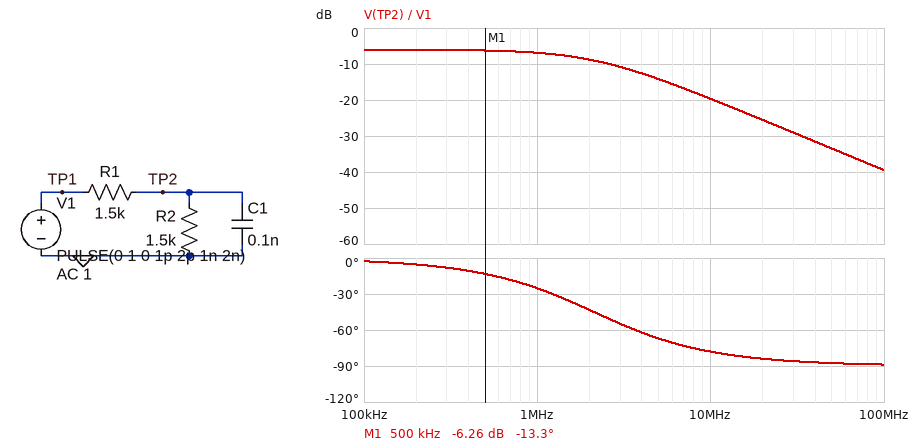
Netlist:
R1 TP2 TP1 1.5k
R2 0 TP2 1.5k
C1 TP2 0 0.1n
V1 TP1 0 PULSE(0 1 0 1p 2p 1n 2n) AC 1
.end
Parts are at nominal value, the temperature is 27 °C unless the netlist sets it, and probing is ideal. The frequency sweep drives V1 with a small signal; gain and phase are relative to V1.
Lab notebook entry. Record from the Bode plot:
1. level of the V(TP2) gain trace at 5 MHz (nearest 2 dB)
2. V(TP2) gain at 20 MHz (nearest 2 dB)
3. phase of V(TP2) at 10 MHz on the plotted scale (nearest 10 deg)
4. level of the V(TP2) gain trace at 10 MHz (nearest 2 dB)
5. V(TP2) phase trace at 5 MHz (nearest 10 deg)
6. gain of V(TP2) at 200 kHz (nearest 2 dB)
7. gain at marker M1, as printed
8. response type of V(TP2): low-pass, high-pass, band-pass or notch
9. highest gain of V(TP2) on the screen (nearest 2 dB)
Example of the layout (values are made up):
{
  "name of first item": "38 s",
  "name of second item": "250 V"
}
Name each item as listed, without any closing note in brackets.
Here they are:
{
  "level of the V(TP2) gain trace at 5 MHz": "-14 dB",
  "V(TP2) gain at 20 MHz": "-26 dB",
  "phase of V(TP2) at 10 MHz on the plotted scale": "-80 deg",
  "level of the V(TP2) gain trace at 10 MHz": "-20 dB",
  "V(TP2) phase trace at 5 MHz": "-70 deg",
  "gain of V(TP2) at 200 kHz": "-6 dB",
  "gain at marker M1, as printed": "-6.26 dB",
  "response type of V(TP2): low-pass, high-pass, band-pass or notch": "low-pass",
  "highest gain of V(TP2) on the screen": "-6 dB"
}
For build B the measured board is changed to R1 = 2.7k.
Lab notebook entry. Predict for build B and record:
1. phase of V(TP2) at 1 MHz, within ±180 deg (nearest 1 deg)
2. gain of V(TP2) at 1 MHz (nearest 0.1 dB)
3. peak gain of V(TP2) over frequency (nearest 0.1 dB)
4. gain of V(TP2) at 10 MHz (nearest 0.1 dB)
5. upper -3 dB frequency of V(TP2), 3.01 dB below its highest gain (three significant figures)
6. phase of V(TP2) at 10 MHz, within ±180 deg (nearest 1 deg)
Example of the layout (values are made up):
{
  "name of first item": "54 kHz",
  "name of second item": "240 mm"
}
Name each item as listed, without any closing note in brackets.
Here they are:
{
  "phase of V(TP2) at 1 MHz, within ±180 deg": "-31 deg",
  "gain of V(TP2) at 1 MHz": "-10.3 dB",
  "peak gain of V(TP2) over frequency": "-8.9 dB",
  "gain of V(TP2) at 10 MHz": "-24.7 dB",
  "upper -3 dB frequency of V(TP2), 3.01 dB below its highest gain": "1.65 MHz",
  "phase of V(TP2) at 10 MHz, within ±180 deg": "-81 deg"
}
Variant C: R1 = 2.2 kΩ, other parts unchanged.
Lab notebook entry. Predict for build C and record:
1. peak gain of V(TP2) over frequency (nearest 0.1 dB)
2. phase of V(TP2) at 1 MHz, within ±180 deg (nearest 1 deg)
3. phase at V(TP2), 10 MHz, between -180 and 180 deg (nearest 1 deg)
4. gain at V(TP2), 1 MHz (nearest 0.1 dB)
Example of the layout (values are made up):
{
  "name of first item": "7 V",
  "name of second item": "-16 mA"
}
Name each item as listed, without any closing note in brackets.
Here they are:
{
  "peak gain of V(TP2) over frequency": "-7.8 dB",
  "phase of V(TP2) at 1 MHz, within ±180 deg": "-29 deg",
  "phase at V(TP2), 10 MHz, between -180 and 180 deg": "-80 deg",
  "gain at V(TP2), 1 MHz": "-9.0 dB"
}
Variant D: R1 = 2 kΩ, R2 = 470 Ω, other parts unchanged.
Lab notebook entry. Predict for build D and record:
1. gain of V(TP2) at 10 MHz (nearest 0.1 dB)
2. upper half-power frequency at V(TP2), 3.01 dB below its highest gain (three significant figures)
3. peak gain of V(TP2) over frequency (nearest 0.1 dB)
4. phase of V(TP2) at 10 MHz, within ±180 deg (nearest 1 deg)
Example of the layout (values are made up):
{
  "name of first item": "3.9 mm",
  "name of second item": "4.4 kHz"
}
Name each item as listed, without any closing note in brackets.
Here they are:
{
  "gain of V(TP2) at 10 MHz": "-22.7 dB",
  "upper half-power frequency at V(TP2), 3.01 dB below its highest gain": "4.18 MHz",
  "peak gain of V(TP2) over frequency": "-14.4 dB",
  "phase of V(TP2) at 10 MHz, within ±180 deg": "-67 deg"
}
